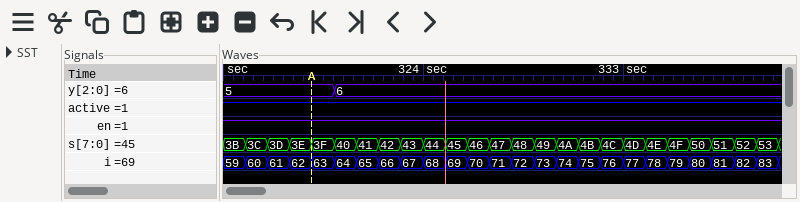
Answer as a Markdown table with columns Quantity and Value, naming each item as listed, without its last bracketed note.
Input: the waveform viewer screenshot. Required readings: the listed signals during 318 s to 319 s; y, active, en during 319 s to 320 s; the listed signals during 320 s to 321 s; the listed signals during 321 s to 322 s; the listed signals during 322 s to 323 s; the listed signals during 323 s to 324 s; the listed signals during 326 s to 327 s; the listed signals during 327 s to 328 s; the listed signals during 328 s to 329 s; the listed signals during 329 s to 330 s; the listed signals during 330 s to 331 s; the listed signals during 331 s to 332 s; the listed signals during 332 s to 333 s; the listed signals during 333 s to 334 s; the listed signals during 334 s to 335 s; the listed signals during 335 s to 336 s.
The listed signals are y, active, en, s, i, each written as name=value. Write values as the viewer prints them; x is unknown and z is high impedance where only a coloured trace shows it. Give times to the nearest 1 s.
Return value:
| Quantity | Value |
|---|---|
| the listed signals during 318 s to 319 s | y=5, active=1, en=1, s=3E, i=62 |
| y, active, en during 319 s to 320 s | y=5, active=1, en=1 |
| the listed signals during 320 s to 321 s | y=6, active=1, en=1, s=40, i=64 |
| the listed signals during 321 s to 322 s | y=6, active=1, en=1, s=41, i=65 |
| the listed signals during 322 s to 323 s | y=6, active=1, en=1, s=42, i=66 |
| the listed signals during 323 s to 324 s | y=6, active=1, en=1, s=43, i=67 |
| the listed signals during 326 s to 327 s | y=6, active=1, en=1, s=46, i=70 |
| the listed signals during 327 s to 328 s | y=6, active=1, en=1, s=47, i=71 |
| the listed signals during 328 s to 329 s | y=6, active=1, en=1, s=48, i=72 |
| the listed signals during 329 s to 330 s | y=6, active=1, en=1, s=49, i=73 |
| the listed signals during 330 s to 331 s | y=6, active=1, en=1, s=4A, i=74 |
| the listed signals during 331 s to 332 s | y=6, active=1, en=1, s=4B, i=75 |
| the listed signals during 332 s to 333 s | y=6, active=1, en=1, s=4C, i=76 |
| the listed signals during 333 s to 334 s | y=6, active=1, en=1, s=4D, i=77 |
| the listed signals during 334 s to 335 s | y=6, active=1, en=1, s=4E, i=78 |
| the listed signals during 335 s to 336 s | y=6, active=1, en=1, s=4F, i=79 |
